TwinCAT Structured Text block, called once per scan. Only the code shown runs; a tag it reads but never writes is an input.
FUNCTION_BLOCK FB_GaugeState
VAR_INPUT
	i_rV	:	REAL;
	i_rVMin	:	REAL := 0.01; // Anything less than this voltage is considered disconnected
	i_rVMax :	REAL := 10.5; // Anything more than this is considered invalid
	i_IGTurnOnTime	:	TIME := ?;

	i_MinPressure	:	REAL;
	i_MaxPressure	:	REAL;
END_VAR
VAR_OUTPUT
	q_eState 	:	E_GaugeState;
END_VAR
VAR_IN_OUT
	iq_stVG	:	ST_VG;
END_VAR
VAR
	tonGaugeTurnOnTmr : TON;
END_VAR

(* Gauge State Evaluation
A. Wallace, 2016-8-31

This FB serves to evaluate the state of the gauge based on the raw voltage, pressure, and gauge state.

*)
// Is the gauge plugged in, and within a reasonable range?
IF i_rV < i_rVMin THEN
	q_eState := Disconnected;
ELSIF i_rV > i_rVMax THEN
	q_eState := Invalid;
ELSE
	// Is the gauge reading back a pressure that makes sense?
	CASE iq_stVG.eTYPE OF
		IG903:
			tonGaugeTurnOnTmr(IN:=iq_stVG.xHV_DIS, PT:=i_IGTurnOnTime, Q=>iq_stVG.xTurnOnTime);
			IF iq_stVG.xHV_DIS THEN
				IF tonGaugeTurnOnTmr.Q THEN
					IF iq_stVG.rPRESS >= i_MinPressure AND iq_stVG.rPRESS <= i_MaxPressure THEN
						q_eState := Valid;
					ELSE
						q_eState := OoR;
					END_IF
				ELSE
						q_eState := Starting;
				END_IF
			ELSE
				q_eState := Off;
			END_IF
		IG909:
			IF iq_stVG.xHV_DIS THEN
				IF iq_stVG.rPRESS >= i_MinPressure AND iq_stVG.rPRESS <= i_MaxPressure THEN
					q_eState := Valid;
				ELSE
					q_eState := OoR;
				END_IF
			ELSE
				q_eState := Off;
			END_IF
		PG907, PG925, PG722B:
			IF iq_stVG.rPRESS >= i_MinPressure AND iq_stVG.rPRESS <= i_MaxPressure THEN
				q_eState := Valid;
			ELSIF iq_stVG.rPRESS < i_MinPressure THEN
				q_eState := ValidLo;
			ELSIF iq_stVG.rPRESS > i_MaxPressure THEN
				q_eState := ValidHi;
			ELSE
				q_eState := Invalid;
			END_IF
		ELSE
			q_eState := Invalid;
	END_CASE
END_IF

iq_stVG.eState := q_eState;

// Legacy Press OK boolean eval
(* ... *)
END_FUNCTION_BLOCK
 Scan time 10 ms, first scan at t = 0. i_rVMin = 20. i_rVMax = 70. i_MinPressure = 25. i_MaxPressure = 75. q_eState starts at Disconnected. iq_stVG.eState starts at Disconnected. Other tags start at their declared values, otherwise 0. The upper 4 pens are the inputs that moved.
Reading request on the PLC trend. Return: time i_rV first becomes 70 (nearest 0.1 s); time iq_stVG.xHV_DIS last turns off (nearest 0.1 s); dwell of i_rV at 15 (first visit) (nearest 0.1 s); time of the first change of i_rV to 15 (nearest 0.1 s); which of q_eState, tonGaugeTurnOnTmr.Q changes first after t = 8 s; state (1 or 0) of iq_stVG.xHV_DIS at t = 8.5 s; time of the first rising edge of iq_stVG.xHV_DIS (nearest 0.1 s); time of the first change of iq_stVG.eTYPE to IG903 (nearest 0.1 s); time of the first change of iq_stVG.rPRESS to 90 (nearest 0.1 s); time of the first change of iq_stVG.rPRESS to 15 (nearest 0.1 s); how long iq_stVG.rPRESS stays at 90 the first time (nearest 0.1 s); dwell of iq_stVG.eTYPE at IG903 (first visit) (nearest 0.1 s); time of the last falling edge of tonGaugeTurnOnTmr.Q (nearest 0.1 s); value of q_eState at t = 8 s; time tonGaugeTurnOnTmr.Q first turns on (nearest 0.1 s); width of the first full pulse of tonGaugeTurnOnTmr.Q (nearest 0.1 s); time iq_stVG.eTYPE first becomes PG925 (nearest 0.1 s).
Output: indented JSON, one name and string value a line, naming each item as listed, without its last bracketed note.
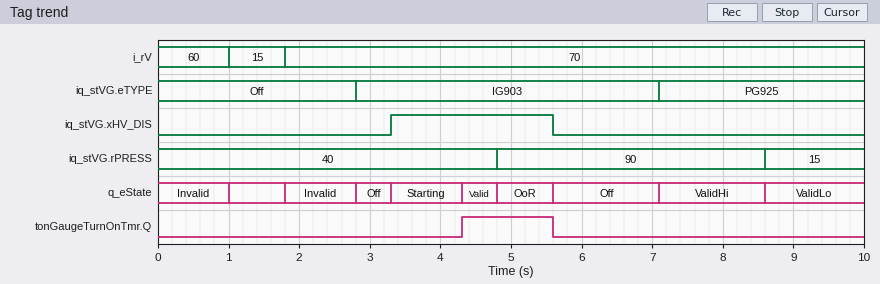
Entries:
{
  "time i_rV first becomes 70": "1.8 s",
  "time iq_stVG.xHV_DIS last turns off": "5.6 s",
  "dwell of i_rV at 15 (first visit)": "0.8 s",
  "time of the first change of i_rV to 15": "1.0 s",
  "which of q_eState, tonGaugeTurnOnTmr.Q changes first after t = 8 s": "q_eState",
  "state (1 or 0) of iq_stVG.xHV_DIS at t = 8.5 s": "0",
  "time of the first rising edge of iq_stVG.xHV_DIS": "3.3 s",
  "time of the first change of iq_stVG.eTYPE to IG903": "2.8 s",
  "time of the first change of iq_stVG.rPRESS to 90": "4.8 s",
  "time of the first change of iq_stVG.rPRESS to 15": "8.6 s",
  "how long iq_stVG.rPRESS stays at 90 the first time": "3.8 s",
  "dwell of iq_stVG.eTYPE at IG903 (first visit)": "4.3 s",
  "time of the last falling edge of tonGaugeTurnOnTmr.Q": "5.6 s",
  "value of q_eState at t = 8 s": "ValidHi",
  "time tonGaugeTurnOnTmr.Q first turns on": "4.3 s",
  "width of the first full pulse of tonGaugeTurnOnTmr.Q": "1.3 s",
  "time iq_stVG.eTYPE first becomes PG925": "7.1 s"
}
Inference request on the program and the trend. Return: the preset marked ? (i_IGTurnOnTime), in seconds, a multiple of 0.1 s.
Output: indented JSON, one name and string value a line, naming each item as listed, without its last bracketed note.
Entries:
{
  "the preset marked ? (i_IGTurnOnTime), in seconds, a multiple of 0.1 s": "1.0 s"
}
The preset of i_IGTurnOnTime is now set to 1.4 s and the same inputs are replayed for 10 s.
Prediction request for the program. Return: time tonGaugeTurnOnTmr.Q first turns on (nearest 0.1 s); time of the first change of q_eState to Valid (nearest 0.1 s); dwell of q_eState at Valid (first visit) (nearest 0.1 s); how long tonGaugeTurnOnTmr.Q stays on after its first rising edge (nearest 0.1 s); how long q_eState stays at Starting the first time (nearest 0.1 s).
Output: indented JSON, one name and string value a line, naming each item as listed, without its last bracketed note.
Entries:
{
  "time tonGaugeTurnOnTmr.Q first turns on": "4.7 s",
  "time of the first change of q_eState to Valid": "4.7 s",
  "dwell of q_eState at Valid (first visit)": "0.1 s",
  "how long tonGaugeTurnOnTmr.Q stays on after its first rising edge": "0.9 s",
  "how long q_eState stays at Starting the first time": "1.4 s"
}
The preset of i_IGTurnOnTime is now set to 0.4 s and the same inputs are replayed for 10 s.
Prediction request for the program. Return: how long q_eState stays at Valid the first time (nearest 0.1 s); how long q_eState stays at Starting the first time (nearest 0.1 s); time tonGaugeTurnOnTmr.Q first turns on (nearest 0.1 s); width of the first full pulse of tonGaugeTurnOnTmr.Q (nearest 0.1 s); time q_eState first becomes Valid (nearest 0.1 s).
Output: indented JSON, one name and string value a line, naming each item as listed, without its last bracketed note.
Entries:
{
  "how long q_eState stays at Valid the first time": "1.1 s",
  "how long q_eState stays at Starting the first time": "0.4 s",
  "time tonGaugeTurnOnTmr.Q first turns on": "3.7 s",
  "width of the first full pulse of tonGaugeTurnOnTmr.Q": "1.9 s",
  "time q_eState first becomes Valid": "3.7 s"
}
